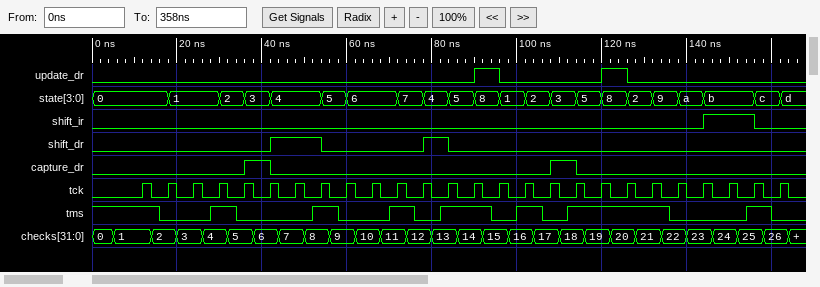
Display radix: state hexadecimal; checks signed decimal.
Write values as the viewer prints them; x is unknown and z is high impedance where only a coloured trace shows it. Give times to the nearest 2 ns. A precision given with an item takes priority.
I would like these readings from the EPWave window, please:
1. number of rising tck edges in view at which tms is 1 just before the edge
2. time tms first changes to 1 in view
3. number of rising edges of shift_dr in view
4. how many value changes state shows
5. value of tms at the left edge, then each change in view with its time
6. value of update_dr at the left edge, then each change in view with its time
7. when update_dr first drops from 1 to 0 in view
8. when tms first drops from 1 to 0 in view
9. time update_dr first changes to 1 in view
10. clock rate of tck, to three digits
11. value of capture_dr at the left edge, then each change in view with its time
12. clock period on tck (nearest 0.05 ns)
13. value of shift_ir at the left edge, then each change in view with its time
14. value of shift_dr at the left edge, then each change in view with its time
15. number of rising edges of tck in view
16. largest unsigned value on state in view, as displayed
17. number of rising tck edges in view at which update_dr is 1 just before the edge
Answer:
12
28 ns
2
21
1, 0 at 16 ns, 1 at 28 ns, 0 at 34 ns, 1 at 52 ns, 0 at 58 ns, 1 at 70 ns, 0 at 76 ns, 1 at 82 ns, 0 at 94 ns, 1 at 100 ns, 0 at 106 ns, 1 at 112 ns, 0 at 136 ns, 1 at 154 ns, 0 at 160 ns
0, 1 at 90 ns, 0 at 96 ns, 1 at 120 ns, 0 at 126 ns
96 ns
16 ns
90 ns
167 MHz
0, 1 at 36 ns, 0 at 42 ns, 1 at 108 ns, 0 at 114 ns
6 ns
0, 1 at 144 ns, 0 at 156 ns
0, 1 at 42 ns, 0 at 54 ns, 1 at 78 ns, 0 at 84 ns
26
d
2
